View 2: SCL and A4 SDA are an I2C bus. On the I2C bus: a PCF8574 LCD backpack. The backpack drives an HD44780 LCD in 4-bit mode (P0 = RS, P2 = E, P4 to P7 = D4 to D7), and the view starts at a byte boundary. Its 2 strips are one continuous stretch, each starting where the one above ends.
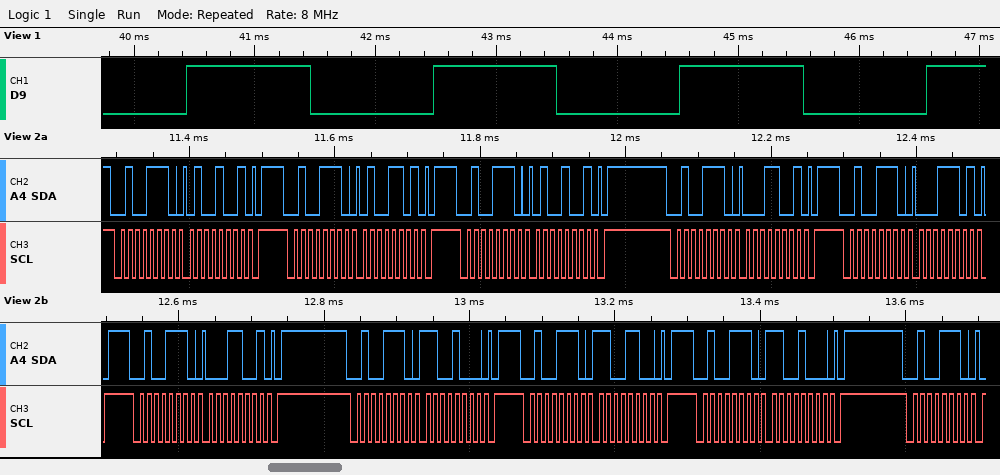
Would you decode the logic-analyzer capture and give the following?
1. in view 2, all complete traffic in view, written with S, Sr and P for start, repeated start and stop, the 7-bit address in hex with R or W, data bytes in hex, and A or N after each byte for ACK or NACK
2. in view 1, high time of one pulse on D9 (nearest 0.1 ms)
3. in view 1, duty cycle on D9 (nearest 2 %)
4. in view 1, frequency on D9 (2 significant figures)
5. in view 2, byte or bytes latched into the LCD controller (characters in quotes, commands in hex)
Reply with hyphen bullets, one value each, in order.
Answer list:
- S 27W A 49 A P S 27W A 4D A P S 27W A 49 A P S 27W A 19 A P S 27W A 1D A P S 27W A 19 A P S 27W A C8 A P S 27W A CC A P S 27W A C8 A P S 27W A
- 1.0 ms
- 50 %
- 490 Hz
- 'A'
